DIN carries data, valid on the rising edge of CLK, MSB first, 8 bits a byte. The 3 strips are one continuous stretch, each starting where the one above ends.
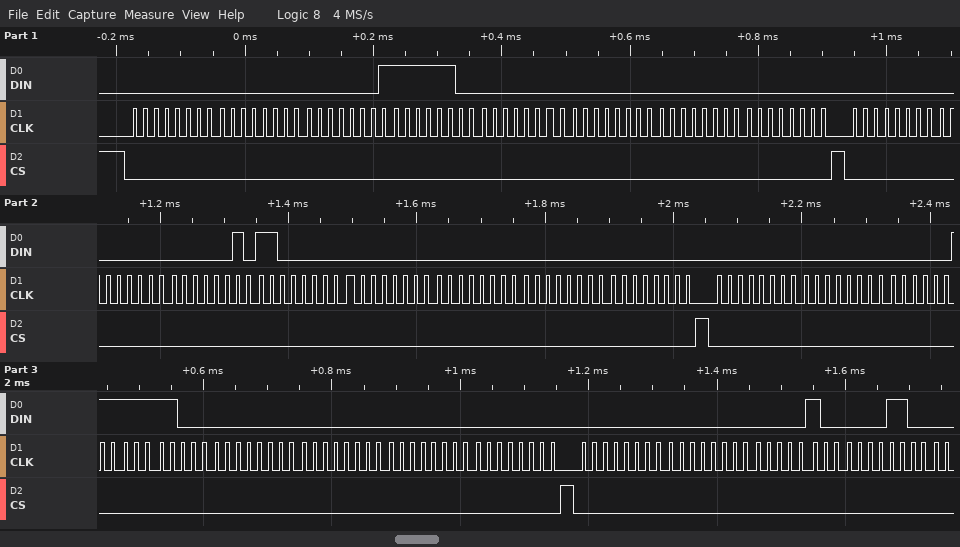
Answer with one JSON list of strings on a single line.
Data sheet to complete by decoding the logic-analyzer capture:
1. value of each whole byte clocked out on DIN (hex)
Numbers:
["00 00 01 FC 00 00 00 00 00 00 02 C0 00 00 00 00 00 00 03 F8 00 00 00 00 00 00 04 0C"]
